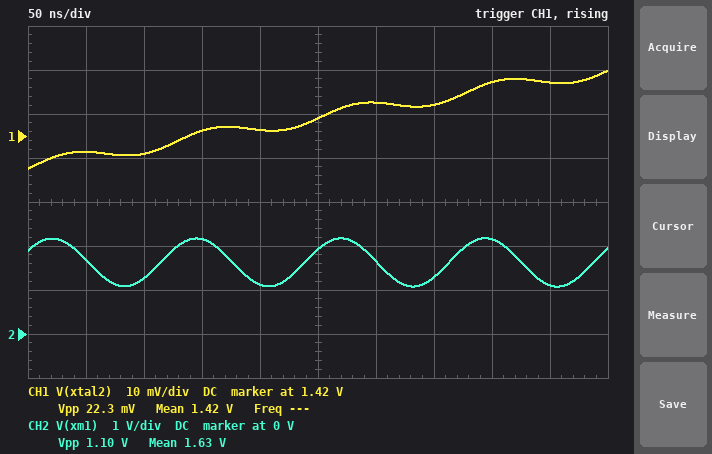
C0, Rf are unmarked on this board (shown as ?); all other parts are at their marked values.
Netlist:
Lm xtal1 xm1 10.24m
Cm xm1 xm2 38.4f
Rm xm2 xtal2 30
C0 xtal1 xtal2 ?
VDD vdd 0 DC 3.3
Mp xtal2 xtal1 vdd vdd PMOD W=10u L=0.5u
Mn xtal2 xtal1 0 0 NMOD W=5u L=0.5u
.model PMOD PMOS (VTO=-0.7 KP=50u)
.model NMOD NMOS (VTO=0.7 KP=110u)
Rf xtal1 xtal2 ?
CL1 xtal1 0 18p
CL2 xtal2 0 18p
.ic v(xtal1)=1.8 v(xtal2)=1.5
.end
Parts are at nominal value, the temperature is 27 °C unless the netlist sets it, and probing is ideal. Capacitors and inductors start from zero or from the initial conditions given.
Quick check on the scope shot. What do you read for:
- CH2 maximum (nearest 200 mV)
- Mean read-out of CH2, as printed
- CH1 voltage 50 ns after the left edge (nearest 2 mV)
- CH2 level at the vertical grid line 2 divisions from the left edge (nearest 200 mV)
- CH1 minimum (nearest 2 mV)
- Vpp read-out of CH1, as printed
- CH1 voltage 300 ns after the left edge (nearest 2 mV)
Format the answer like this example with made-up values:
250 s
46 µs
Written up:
2.2 V
1.63 V
1.416 V
1.2 V
1.412 V
22.3 mV
1.428 V
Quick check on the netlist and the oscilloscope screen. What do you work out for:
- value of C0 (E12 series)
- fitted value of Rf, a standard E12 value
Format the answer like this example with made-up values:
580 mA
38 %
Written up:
5.6 pF
820 kΩ
